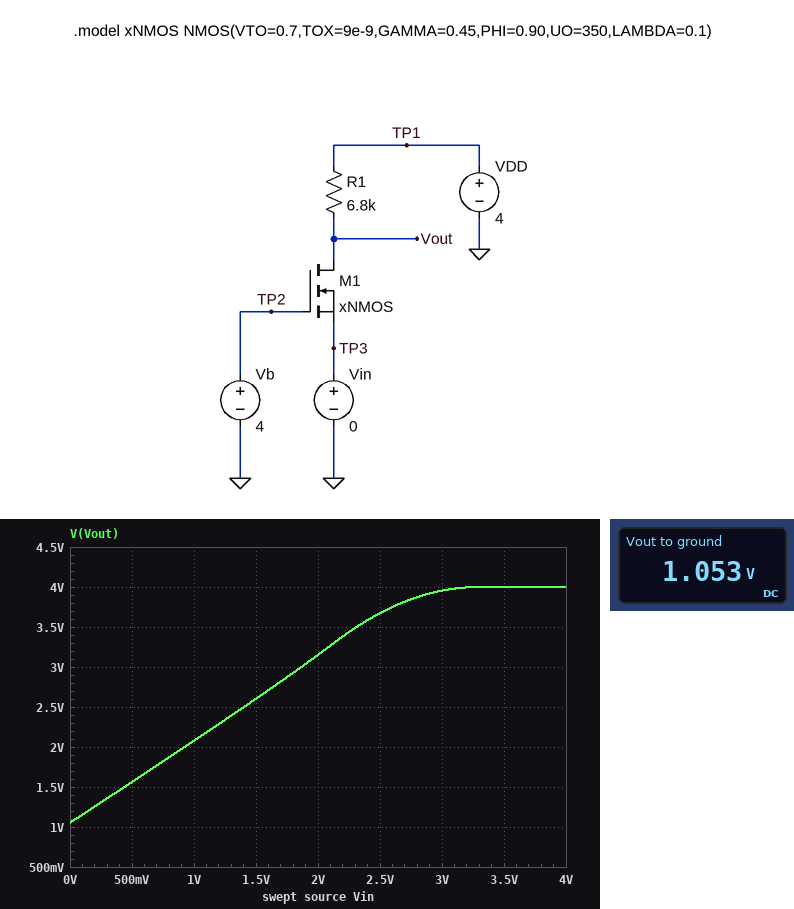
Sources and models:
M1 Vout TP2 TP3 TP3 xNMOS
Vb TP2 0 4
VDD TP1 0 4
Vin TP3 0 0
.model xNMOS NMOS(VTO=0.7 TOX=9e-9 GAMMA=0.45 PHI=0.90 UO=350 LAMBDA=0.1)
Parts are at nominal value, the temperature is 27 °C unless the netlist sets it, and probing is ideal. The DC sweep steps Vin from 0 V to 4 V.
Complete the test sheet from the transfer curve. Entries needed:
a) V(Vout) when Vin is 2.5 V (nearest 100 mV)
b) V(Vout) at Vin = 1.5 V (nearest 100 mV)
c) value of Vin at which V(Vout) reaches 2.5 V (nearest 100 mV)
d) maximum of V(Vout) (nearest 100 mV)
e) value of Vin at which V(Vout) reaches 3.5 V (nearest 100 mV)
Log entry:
3.7 V
2.6 V
1.4 V
4.0 V
2.3 V
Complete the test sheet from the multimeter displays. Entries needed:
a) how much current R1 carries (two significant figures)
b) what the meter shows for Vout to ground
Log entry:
430 µA
1.053 V
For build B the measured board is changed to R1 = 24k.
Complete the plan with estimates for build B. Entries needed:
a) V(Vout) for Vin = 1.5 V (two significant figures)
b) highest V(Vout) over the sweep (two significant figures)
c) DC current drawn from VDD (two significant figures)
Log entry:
1.9 V
4.0 V
150 µA
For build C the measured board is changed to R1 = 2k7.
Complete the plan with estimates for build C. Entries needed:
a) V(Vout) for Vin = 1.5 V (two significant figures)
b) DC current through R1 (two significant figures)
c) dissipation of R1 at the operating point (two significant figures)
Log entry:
3.3 V
740 µA
1.5 mW
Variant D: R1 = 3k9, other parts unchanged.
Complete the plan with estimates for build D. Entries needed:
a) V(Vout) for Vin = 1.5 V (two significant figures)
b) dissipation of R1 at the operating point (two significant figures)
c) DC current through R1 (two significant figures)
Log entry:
3.0 V
1.5 mW
620 µA
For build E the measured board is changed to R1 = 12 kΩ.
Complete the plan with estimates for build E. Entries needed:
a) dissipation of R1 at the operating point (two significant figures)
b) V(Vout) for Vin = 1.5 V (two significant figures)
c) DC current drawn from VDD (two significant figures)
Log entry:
930 µW
2.2 V
280 µA
